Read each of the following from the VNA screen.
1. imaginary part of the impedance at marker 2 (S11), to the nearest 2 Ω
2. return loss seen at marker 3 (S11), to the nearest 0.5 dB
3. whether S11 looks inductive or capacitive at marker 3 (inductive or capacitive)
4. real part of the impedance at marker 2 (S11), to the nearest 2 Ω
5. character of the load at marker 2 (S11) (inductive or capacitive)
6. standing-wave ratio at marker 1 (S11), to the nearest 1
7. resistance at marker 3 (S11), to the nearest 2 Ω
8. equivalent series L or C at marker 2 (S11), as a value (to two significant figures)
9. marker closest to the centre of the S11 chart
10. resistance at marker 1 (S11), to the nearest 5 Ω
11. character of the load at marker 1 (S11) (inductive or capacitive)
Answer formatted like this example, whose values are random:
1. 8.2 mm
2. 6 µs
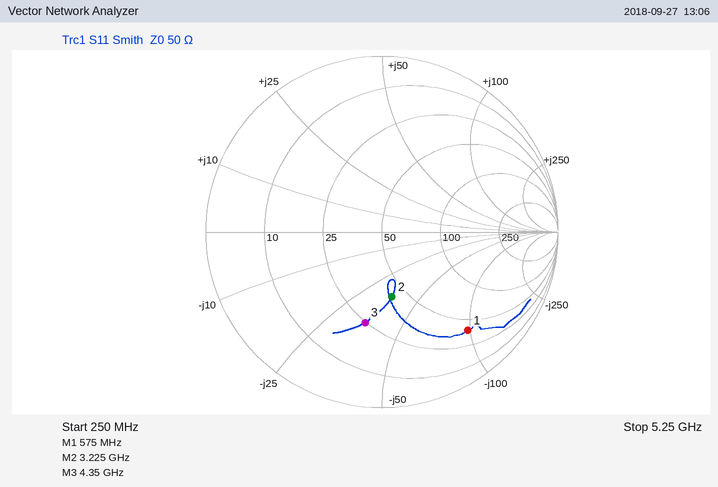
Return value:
1. -36 Ω
2. 5.5 dB
3. capacitive
4. 42 Ω
5. capacitive
6. 7
7. 24 Ω
8. 1.4 pF
9. marker 2
10. 40 Ω
11. capacitive
